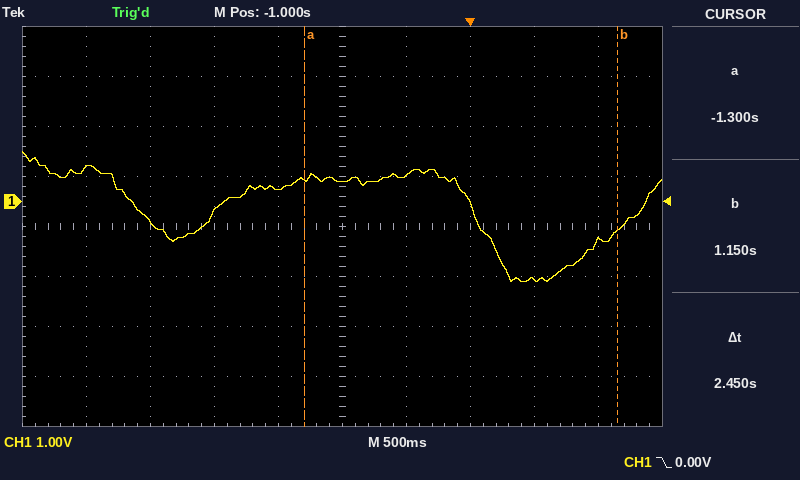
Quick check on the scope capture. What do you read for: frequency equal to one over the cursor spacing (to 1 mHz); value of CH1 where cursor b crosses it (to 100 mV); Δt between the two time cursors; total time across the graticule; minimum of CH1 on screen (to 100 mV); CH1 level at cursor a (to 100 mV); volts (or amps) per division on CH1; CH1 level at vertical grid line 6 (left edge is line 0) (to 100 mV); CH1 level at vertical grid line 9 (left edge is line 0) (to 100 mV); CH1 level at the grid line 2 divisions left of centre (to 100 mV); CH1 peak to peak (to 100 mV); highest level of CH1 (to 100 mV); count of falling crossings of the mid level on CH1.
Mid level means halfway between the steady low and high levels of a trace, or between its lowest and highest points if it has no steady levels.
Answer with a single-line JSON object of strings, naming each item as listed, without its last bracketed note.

{"frequency equal to one over the cursor spacing": "408 mHz", "value of CH1 where cursor b crosses it": "-600 mV", "Δt between the two time cursors": "2.45 s", "total time across the graticule": "5 s", "minimum of CH1 on screen": "-1.6 V", "CH1 level at cursor a": "400 mV", "volts (or amps) per division on CH1": "1 V", "CH1 level at vertical grid line 6 (left edge is line 0)": "500 mV", "CH1 level at vertical grid line 9 (left edge is line 0)": "-800 mV", "CH1 level at the grid line 2 divisions left of centre": "-200 mV", "CH1 peak to peak": "2.6 V", "highest level of CH1": "1.0 V", "count of falling crossings of the mid level on CH1": "2"}
